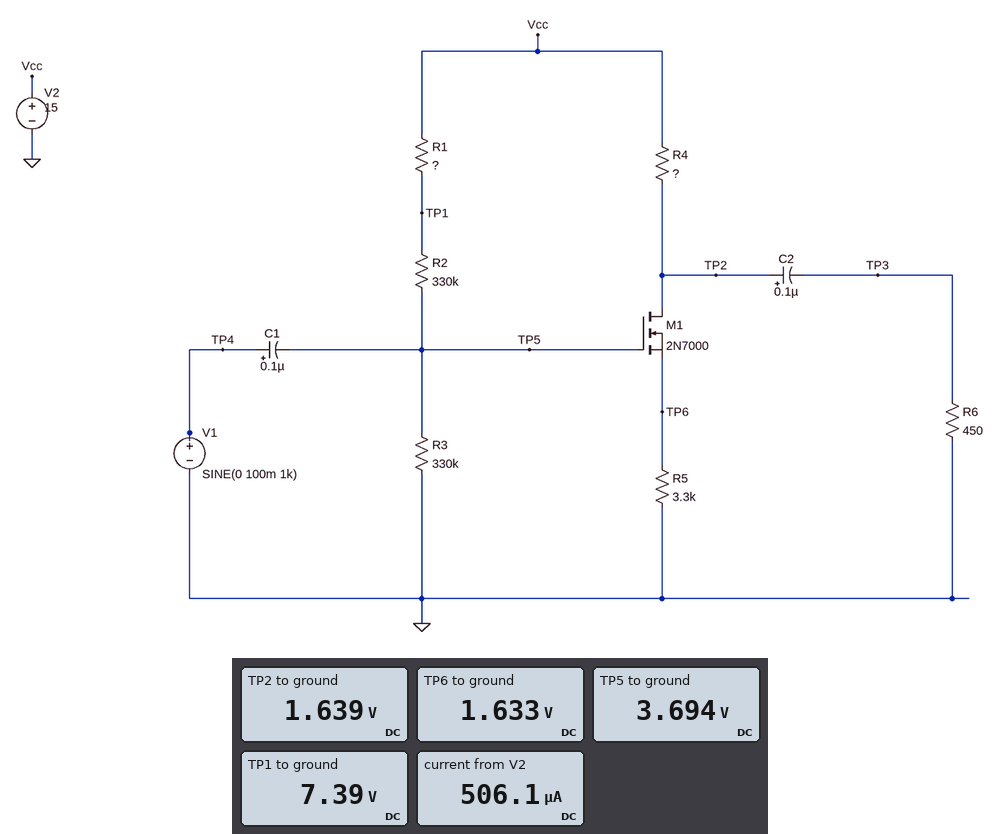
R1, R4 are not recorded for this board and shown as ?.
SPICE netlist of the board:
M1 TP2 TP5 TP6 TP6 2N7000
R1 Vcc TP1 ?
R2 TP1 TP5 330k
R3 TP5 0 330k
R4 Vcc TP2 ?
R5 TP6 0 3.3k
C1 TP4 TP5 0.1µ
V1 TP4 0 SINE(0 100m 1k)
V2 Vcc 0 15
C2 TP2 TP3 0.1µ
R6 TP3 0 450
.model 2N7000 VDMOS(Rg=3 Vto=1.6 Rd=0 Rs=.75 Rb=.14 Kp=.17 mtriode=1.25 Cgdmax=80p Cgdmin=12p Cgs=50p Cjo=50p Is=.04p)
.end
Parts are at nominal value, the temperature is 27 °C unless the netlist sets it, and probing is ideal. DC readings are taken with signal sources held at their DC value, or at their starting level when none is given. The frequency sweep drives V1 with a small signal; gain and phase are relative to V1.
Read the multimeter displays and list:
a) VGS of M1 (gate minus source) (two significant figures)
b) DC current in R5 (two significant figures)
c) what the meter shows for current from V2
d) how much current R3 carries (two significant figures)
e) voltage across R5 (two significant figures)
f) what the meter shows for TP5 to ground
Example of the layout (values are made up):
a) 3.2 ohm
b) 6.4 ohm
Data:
a) 2.1 V
b) 490 µA
c) 506.1 µA
d) 11 µA
e) 1.6 V
f) 3.694 V
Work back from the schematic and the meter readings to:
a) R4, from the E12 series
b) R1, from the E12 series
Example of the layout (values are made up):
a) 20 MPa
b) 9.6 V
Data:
a) 27 kΩ
b) 680 kΩ
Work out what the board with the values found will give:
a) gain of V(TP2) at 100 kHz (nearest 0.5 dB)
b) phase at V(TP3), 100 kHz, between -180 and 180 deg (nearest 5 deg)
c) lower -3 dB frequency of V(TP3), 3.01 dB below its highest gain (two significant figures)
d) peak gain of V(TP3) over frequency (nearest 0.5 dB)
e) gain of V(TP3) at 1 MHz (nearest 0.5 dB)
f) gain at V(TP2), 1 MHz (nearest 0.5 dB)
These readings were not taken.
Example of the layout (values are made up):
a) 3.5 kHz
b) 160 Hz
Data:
a) -30.0 dB
b) 90 deg
c) 3.2 MHz
d) 0 dB
e) -10.5 dB
f) -10.5 dB
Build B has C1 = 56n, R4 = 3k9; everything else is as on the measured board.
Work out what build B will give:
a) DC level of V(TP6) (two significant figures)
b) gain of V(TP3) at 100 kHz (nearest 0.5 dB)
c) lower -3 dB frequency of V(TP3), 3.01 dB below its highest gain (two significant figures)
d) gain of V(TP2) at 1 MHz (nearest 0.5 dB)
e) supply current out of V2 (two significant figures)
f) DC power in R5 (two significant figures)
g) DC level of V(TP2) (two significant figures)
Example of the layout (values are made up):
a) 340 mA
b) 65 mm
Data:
a) 2.1 V
b) -18.5 dB
c) 14 MHz
d) -18.0 dB
e) 640 µA
f) 1.3 mW
g) 13 V
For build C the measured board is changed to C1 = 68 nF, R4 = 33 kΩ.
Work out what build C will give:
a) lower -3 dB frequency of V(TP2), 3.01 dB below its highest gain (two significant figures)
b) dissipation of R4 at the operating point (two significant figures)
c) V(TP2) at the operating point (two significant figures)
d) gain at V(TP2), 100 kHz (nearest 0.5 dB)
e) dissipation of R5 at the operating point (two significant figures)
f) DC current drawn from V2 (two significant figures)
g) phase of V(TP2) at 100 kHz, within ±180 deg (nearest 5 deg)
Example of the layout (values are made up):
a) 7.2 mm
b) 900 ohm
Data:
a) 3.1 MHz
b) 5.6 mW
c) 1.4 V
d) -30.0 dB
e) 560 µW
f) 420 µA
g) 85 deg
